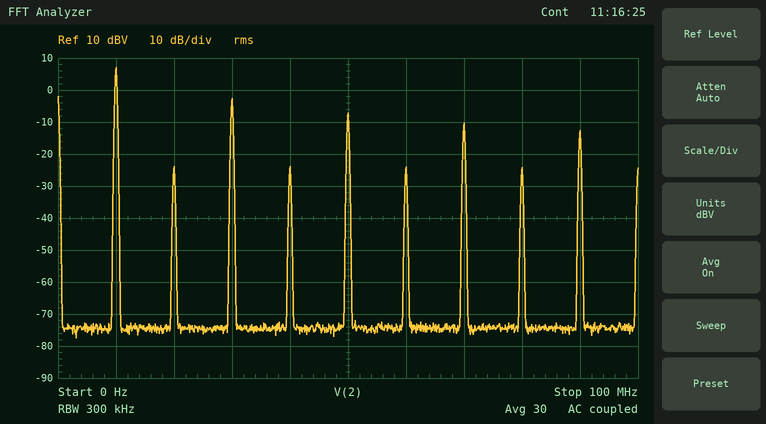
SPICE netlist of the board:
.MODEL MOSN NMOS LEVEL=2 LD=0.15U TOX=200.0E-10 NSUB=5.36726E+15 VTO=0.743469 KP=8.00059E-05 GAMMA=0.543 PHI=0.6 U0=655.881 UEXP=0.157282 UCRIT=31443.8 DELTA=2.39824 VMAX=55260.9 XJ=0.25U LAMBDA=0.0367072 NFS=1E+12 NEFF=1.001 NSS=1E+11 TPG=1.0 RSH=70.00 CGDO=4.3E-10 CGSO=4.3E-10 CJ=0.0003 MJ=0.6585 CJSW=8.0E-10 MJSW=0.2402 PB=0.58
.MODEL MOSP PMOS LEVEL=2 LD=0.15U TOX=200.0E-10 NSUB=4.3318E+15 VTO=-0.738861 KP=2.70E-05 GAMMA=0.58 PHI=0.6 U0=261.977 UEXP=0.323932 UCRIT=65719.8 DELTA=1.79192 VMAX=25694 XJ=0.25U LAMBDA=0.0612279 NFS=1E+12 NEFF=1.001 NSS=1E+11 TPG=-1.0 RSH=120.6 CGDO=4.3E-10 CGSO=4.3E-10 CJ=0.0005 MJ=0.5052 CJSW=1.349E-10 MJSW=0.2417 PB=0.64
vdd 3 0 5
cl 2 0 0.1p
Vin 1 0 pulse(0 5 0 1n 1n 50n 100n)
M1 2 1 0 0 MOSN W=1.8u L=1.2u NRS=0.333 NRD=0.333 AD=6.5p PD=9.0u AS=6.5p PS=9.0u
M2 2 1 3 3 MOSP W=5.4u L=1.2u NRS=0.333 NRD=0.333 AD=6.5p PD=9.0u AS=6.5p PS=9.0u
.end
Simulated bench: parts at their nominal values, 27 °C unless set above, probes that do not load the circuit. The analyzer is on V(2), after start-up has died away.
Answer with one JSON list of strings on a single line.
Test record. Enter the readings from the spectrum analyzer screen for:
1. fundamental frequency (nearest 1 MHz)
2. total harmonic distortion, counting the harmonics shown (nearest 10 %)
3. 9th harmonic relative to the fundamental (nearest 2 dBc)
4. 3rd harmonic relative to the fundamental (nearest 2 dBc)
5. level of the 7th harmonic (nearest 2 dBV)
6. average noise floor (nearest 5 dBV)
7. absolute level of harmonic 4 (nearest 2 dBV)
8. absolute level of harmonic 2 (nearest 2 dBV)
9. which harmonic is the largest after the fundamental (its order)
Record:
["10 MHz", "40 %", "-20 dBc", "-10 dBc", "-10 dBV", "-75 dBV", "-24 dBV", "-24 dBV", "3"]
